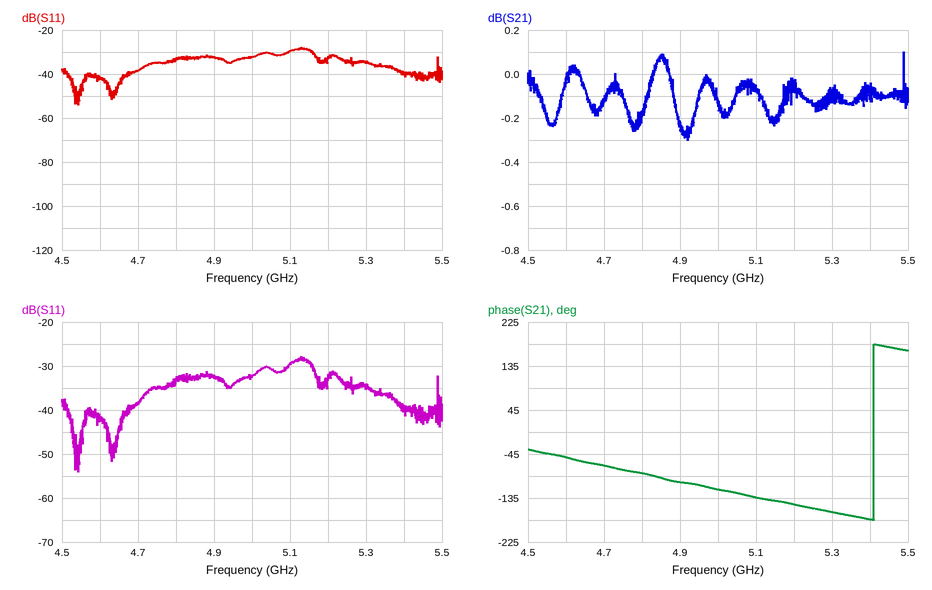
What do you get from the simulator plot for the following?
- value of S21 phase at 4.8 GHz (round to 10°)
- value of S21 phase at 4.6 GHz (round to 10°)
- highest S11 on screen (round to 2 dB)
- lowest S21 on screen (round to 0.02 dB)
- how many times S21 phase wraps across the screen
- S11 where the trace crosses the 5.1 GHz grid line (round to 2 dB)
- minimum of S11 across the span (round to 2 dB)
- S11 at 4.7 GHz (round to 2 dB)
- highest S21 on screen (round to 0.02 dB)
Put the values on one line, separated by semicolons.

-80°; -50°; -28 dB; -0.30 dB; 1; -30 dB; -54 dB; -38 dB; 0.10 dB
